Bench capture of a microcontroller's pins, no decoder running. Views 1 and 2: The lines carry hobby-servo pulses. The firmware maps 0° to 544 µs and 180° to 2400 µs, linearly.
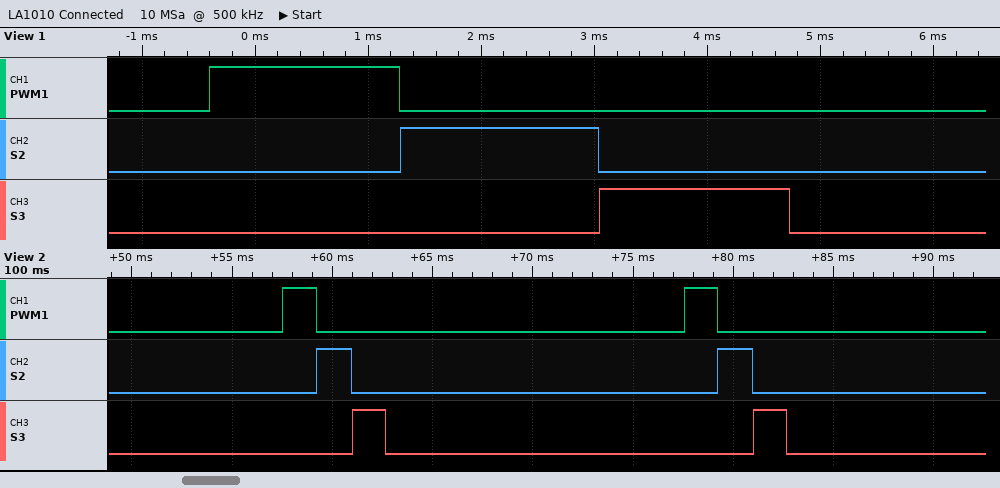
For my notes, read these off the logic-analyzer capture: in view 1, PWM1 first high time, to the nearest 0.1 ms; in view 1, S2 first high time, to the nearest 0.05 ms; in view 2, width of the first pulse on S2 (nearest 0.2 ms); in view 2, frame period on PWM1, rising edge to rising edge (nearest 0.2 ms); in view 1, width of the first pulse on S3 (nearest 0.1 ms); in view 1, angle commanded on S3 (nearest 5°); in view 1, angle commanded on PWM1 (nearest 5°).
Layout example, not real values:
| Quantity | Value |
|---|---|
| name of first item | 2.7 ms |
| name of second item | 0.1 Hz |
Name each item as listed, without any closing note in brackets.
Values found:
| Quantity | Value |
|---|---|
| in view 1, PWM1 first high time, to the nearest 0.1 ms | 1.7 ms |
| in view 1, S2 first high time, to the nearest 0.05 ms | 1.75 ms |
| in view 2, width of the first pulse on S2 | 1.8 ms |
| in view 2, frame period on PWM1, rising edge to rising edge | 20.0 ms |
| in view 1, width of the first pulse on S3 | 1.7 ms |
| in view 1, angle commanded on S3 | 110° |
| in view 1, angle commanded on PWM1 | 110° |
